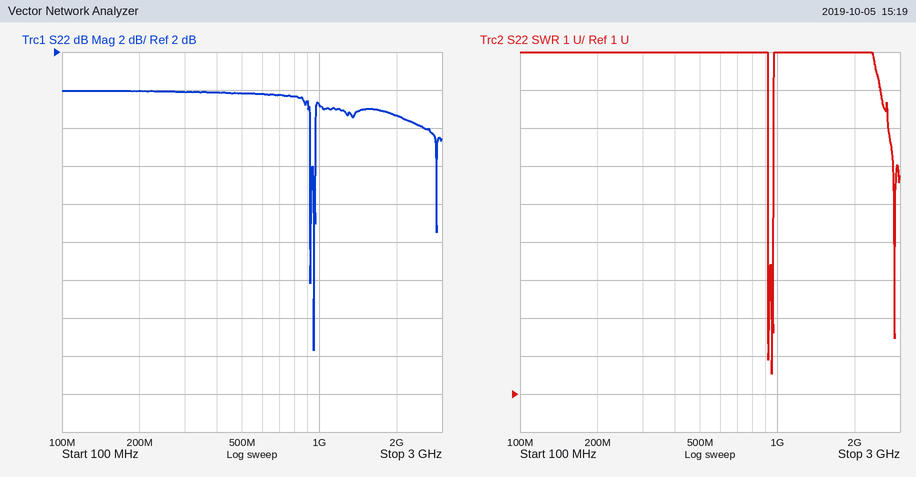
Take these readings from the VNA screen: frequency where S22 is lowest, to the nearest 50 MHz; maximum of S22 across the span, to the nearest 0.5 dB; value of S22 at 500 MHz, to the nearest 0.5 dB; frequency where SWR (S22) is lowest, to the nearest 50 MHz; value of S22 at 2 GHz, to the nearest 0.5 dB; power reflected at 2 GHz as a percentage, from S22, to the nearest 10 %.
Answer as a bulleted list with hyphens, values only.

- 950 MHz
- 0.0 dB
- 0.0 dB
- 950 MHz
- -1.5 dB
- 70 %
